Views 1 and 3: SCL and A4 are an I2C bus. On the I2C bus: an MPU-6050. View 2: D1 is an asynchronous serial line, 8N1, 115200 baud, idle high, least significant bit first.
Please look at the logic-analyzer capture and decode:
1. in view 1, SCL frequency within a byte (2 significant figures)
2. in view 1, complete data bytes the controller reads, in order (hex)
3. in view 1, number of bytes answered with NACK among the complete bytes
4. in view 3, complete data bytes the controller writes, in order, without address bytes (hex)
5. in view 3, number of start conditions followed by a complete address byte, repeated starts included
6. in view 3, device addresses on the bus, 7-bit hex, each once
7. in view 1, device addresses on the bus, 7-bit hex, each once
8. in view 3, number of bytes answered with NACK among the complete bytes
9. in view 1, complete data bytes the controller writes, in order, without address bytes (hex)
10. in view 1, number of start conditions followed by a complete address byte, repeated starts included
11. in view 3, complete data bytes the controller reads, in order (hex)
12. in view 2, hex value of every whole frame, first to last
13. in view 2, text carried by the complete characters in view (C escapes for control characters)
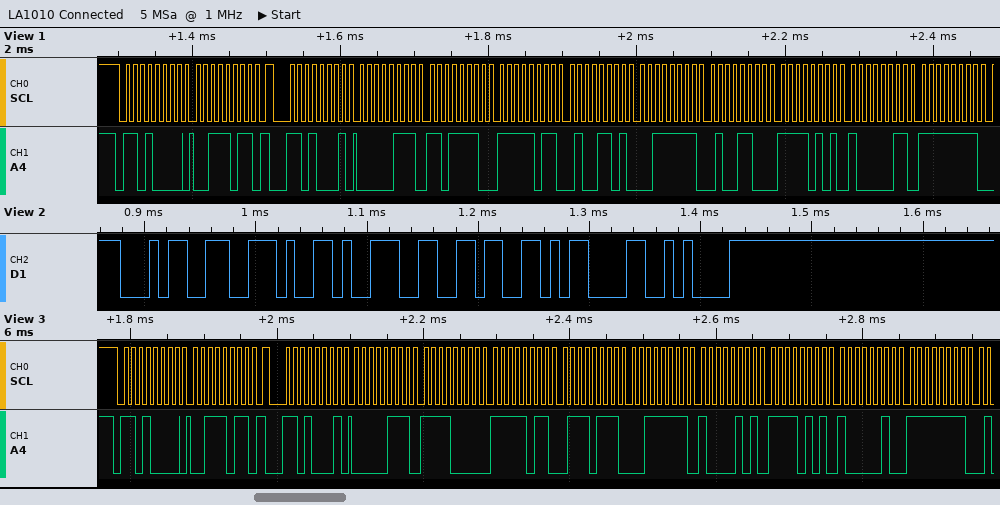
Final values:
100 kHz
07 DE FB 4D 3F 4C F5 83 FF
0
3B
2
0x68
0x68
0
3B
2
07 F0 FB 77 3F 85 F5 82 FF
0x34 0x2E 0x39 0x36 0x0D 0x0A
"4.96\r\n"
